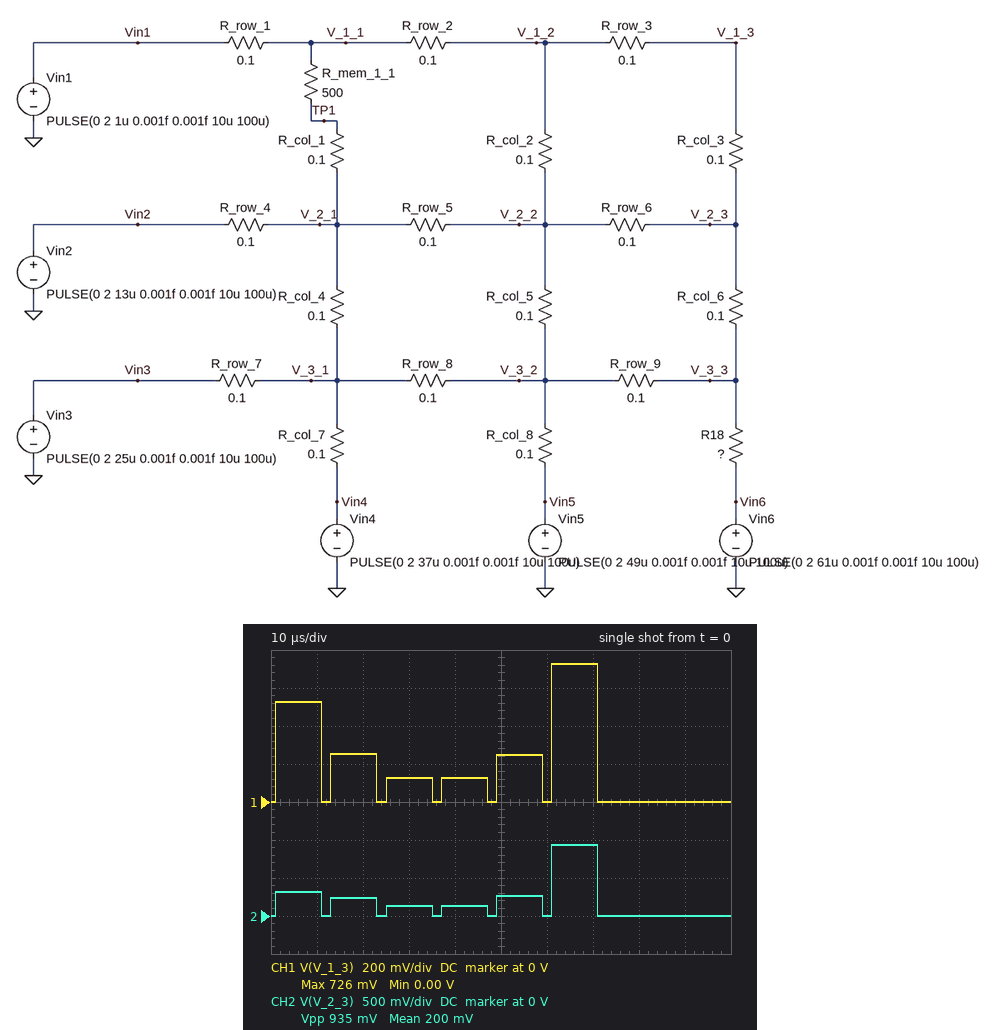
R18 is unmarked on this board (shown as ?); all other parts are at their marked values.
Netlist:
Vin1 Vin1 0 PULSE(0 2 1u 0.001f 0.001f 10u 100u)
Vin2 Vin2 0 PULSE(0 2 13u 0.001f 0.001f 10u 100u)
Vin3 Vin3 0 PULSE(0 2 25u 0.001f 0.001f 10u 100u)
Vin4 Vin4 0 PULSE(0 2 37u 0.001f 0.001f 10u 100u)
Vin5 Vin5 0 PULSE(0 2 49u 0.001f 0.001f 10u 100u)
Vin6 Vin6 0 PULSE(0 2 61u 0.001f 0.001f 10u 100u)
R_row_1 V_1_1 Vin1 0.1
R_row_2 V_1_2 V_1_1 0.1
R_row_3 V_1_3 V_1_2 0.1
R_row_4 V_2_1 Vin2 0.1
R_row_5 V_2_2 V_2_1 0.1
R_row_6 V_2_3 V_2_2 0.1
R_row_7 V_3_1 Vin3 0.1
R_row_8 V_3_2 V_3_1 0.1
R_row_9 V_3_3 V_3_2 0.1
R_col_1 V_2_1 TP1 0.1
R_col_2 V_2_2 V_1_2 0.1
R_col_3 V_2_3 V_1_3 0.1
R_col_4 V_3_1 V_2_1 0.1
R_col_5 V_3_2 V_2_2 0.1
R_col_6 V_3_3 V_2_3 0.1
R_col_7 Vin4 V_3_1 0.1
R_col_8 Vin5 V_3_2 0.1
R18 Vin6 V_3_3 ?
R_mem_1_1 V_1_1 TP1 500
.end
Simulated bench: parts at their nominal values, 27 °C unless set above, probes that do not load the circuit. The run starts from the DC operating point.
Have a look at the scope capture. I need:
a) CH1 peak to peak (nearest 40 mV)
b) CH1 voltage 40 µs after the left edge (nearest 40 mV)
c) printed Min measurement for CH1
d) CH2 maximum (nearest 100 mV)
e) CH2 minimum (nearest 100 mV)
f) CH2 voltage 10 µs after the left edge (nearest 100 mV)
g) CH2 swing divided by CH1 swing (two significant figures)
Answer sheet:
720 mV
120 mV
0.00 V
900 mV
0 V
300 mV
1.3
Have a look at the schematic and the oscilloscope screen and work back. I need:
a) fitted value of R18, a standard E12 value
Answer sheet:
0.033 Ω
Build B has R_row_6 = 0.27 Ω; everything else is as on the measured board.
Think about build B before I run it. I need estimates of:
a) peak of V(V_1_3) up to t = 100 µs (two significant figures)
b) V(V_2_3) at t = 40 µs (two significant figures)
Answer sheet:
780 mV
110 mV
